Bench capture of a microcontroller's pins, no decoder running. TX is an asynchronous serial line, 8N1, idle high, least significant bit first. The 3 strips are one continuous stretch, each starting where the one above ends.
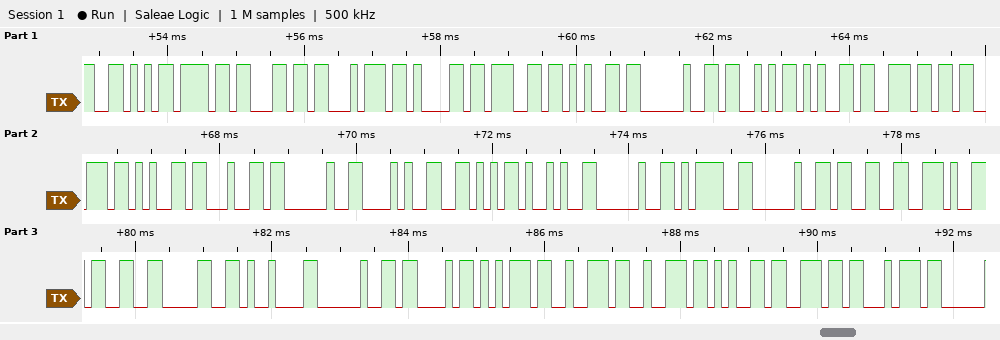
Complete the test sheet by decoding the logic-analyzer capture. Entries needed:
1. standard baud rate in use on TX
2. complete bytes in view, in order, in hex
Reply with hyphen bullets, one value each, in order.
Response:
- 9600 baud
- 56 6F 6C 74 61 67 65 20 53 65 6E 73 65 64 20 28 56 29 20 3D 20 33 2E 33 30 09 20 43 75 72 72 65 6E 74
